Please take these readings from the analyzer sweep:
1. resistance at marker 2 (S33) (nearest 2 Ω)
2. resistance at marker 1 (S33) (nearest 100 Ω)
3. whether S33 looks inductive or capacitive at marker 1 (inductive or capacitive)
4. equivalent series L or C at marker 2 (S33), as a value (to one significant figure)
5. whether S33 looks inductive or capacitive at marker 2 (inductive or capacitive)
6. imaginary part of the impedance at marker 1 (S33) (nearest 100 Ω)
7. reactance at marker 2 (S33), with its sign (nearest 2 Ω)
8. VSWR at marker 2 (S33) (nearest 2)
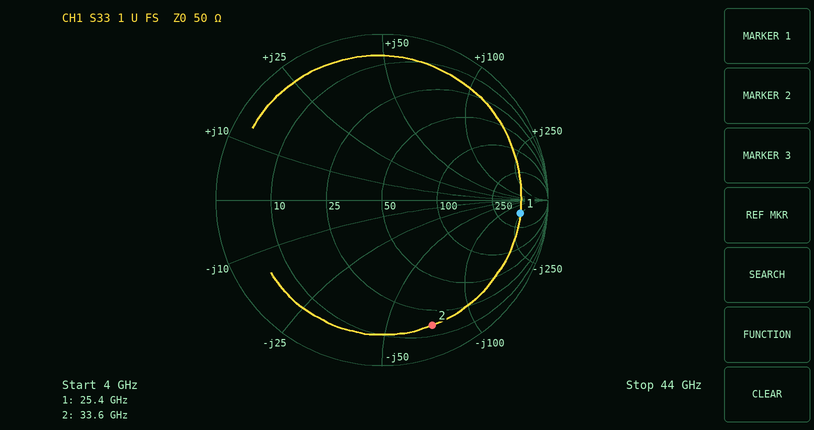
16 Ω
400 Ω
capacitive
70 fF
capacitive
-200 Ω
-72 Ω
10
